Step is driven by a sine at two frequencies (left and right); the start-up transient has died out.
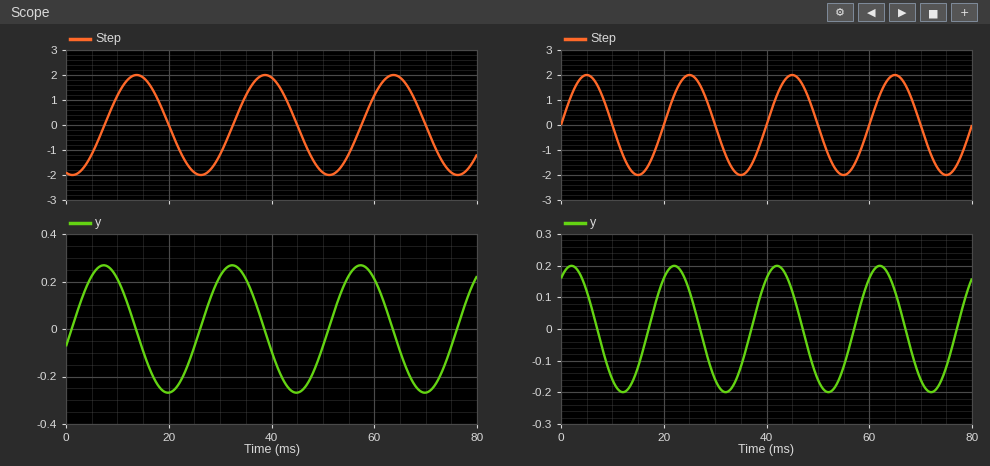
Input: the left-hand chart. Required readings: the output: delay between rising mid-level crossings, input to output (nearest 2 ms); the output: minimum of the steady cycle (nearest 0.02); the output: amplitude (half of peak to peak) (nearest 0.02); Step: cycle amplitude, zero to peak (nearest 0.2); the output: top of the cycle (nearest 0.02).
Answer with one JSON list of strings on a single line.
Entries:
["18 ms", "-0.26", "0.26", "2.0", "0.26"]
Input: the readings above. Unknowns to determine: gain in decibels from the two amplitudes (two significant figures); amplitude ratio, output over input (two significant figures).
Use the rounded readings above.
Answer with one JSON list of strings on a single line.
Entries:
["-18 dB", "0.13"]
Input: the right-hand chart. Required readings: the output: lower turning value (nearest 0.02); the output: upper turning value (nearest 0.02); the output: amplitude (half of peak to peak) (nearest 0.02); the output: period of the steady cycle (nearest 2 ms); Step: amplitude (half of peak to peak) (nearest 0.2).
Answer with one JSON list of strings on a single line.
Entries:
["-0.20", "0.20", "0.20", "20 ms", "2.0"]
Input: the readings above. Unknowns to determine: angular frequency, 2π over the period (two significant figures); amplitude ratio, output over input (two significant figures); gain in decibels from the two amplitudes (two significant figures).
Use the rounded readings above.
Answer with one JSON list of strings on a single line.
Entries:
["0.31 rad/ms", "0.10", "-20 dB"]
